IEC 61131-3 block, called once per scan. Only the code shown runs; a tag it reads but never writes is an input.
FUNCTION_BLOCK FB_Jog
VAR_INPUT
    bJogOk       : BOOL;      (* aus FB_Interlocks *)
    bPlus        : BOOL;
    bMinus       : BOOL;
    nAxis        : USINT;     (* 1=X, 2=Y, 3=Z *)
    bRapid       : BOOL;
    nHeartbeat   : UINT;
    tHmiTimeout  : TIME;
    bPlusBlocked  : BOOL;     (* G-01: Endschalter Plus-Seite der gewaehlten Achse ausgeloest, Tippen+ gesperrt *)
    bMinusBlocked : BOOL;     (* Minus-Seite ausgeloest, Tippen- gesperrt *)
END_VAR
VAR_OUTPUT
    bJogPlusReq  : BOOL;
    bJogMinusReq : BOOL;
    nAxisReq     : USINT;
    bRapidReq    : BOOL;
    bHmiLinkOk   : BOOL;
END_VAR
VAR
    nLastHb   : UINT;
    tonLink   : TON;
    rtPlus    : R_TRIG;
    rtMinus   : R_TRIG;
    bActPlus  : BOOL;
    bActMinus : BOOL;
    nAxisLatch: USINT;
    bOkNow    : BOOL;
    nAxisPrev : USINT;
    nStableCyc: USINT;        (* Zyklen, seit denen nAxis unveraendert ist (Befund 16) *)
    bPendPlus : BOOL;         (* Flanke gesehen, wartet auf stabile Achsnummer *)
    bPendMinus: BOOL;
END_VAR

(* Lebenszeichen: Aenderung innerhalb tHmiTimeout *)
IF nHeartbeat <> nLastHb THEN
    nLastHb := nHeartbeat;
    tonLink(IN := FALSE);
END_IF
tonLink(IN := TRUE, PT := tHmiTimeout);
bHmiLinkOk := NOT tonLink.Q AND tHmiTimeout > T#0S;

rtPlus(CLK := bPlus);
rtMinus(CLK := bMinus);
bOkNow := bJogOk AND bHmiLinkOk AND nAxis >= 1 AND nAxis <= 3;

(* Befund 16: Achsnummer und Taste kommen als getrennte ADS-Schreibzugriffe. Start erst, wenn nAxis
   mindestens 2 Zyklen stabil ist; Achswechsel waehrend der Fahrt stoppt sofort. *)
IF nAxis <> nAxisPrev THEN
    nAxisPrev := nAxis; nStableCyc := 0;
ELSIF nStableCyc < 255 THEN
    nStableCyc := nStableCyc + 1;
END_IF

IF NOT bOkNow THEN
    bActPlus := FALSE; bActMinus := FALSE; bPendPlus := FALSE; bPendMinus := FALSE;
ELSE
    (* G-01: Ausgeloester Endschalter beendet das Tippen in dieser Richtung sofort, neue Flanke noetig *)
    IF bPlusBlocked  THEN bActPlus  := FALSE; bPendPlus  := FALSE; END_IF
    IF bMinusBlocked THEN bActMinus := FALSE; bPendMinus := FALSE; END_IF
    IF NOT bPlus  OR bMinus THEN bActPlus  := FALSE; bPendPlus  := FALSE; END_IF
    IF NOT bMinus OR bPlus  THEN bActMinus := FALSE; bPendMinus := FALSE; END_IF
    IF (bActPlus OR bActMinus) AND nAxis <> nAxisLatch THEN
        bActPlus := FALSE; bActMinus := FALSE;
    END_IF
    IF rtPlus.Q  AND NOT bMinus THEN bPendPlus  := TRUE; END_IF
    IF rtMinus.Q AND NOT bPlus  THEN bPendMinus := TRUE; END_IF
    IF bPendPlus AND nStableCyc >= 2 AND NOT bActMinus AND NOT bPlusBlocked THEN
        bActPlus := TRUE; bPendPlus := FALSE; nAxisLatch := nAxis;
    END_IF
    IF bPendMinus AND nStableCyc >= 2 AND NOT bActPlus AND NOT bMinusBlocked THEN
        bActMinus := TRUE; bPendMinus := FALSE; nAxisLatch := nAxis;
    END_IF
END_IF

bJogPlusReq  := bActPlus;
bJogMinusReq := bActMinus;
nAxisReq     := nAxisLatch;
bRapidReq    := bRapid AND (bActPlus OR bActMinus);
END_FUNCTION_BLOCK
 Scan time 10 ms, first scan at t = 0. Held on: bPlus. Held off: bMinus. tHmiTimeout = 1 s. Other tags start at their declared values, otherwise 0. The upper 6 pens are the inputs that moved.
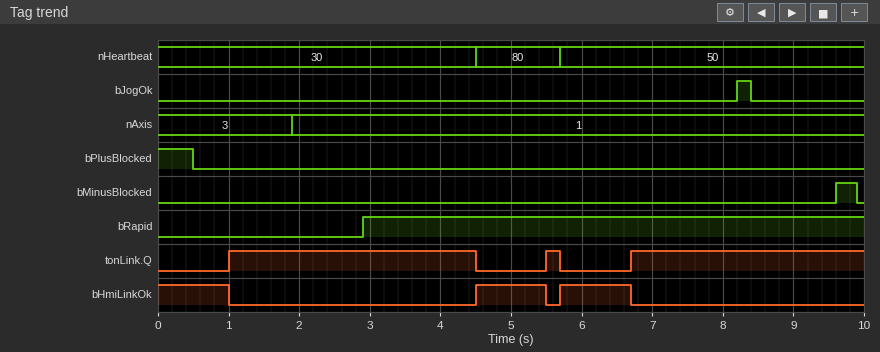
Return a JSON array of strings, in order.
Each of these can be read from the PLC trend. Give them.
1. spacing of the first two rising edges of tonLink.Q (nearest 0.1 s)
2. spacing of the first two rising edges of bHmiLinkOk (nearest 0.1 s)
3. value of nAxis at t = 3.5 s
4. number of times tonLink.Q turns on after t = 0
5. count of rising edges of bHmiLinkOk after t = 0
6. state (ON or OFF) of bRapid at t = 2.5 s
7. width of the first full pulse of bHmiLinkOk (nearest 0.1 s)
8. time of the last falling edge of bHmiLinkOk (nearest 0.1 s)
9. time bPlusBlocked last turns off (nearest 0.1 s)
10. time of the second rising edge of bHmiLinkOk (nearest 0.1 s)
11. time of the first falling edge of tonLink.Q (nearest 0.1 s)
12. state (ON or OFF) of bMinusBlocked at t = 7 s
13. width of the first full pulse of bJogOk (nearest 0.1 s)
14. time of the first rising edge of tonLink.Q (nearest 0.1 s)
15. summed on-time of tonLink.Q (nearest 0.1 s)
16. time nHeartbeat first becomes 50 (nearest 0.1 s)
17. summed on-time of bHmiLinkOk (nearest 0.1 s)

["4.5 s", "1.2 s", "1", "3", "2", "OFF", "1.0 s", "6.7 s", "0.5 s", "5.7 s", "4.5 s", "OFF", "0.2 s", "1.0 s", "7.0 s", "5.7 s", "3.0 s"]
